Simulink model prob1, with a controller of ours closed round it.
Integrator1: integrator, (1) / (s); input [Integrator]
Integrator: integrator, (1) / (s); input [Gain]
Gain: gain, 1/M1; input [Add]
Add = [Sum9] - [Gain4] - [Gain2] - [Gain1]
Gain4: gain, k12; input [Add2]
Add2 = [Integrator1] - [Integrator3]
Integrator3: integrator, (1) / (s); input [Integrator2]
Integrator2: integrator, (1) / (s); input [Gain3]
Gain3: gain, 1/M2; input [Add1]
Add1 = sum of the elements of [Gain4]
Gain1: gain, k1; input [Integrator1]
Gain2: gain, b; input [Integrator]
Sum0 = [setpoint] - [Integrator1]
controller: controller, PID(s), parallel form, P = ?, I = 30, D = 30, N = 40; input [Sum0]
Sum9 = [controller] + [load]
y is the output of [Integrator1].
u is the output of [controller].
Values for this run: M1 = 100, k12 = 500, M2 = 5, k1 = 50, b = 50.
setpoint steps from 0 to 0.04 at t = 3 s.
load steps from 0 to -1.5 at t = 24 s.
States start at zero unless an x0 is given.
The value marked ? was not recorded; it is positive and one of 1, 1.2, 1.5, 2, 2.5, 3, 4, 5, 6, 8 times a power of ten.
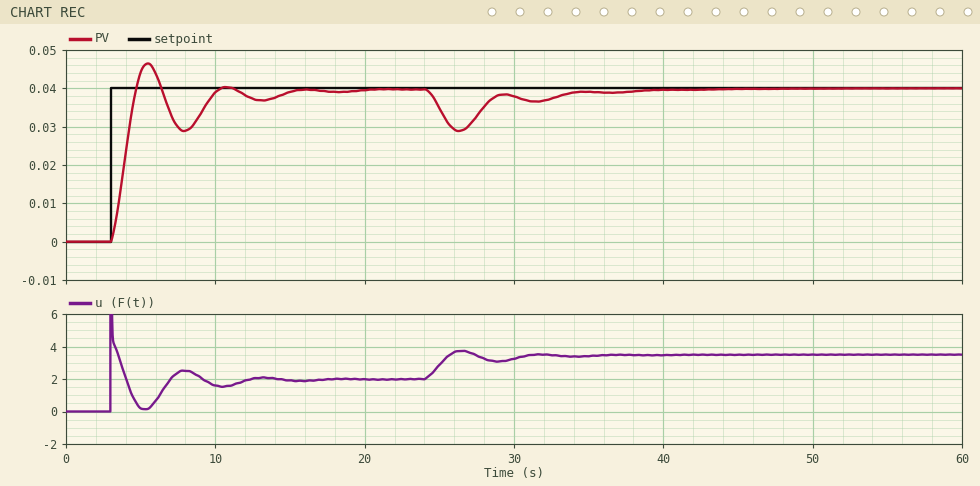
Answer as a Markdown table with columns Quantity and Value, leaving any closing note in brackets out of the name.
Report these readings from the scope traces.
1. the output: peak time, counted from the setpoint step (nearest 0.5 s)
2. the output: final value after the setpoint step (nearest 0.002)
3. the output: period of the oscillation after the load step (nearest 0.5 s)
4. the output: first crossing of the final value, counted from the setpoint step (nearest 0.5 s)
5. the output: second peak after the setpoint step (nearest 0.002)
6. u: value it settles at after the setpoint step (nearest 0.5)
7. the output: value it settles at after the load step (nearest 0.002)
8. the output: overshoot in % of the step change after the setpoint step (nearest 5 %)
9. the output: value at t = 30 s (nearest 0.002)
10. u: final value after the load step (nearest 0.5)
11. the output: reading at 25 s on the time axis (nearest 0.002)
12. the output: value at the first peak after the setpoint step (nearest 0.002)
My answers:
| Quantity | Value |
|---|---|
| the output: peak time, counted from the setpoint step | 2.5 s |
| the output: final value after the setpoint step | 0.040 |
| the output: period of the oscillation after the load step | 5.5 s |
| the output: first crossing of the final value, counted from the setpoint step | 1.5 s |
| the output: second peak after the setpoint step | 0.040 |
| u: value it settles at after the setpoint step | 2.0 |
| the output: value it settles at after the load step | 0.040 |
| the output: overshoot in % of the step change after the setpoint step | 15 % |
| the output: value at t = 30 s | 0.038 |
| u: final value after the load step | 3.5 |
| the output: reading at 25 s on the time axis | 0.034 |
| the output: value at the first peak after the setpoint step | 0.046 |
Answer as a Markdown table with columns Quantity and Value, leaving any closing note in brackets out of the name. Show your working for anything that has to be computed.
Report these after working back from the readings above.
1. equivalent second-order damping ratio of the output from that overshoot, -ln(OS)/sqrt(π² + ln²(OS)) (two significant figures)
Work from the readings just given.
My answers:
| Quantity | Value |
|---|---|
| equivalent second-order damping ratio of the output from that overshoot, -ln(OS)/sqrt(π² + ln²(OS)) | ln(0.15) = -1.897; 1.897 / sqrt(9.870 + 3.599) = 0.52 |
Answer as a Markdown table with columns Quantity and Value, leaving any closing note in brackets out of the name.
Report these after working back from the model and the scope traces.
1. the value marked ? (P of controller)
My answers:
| Quantity | Value |
|---|---|
| the value marked ? | 120 |
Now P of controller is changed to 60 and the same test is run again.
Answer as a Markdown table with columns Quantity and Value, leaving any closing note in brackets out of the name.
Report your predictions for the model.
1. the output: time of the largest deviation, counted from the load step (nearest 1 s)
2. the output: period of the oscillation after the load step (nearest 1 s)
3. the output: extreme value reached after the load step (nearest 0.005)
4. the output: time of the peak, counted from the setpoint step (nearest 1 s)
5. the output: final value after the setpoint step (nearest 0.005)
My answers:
| Quantity | Value |
|---|---|
| the output: time of the largest deviation, counted from the load step | 3 s |
| the output: period of the oscillation after the load step | 7 s |
| the output: extreme value reached after the load step | 0.025 |
| the output: time of the peak, counted from the setpoint step | 3 s |
| the output: final value after the setpoint step | 0.040 |
